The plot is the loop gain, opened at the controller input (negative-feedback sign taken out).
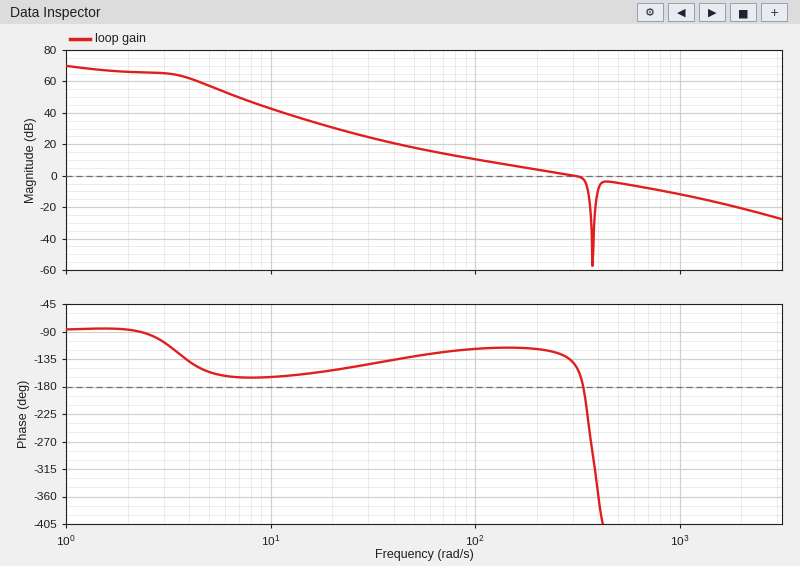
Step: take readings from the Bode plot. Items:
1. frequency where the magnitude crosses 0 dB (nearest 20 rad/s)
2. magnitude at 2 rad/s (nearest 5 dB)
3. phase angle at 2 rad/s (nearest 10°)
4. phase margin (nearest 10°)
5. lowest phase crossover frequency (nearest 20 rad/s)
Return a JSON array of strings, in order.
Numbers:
["300 rad/s", "65 dB", "-90°", "40°", "340 rad/s"]
